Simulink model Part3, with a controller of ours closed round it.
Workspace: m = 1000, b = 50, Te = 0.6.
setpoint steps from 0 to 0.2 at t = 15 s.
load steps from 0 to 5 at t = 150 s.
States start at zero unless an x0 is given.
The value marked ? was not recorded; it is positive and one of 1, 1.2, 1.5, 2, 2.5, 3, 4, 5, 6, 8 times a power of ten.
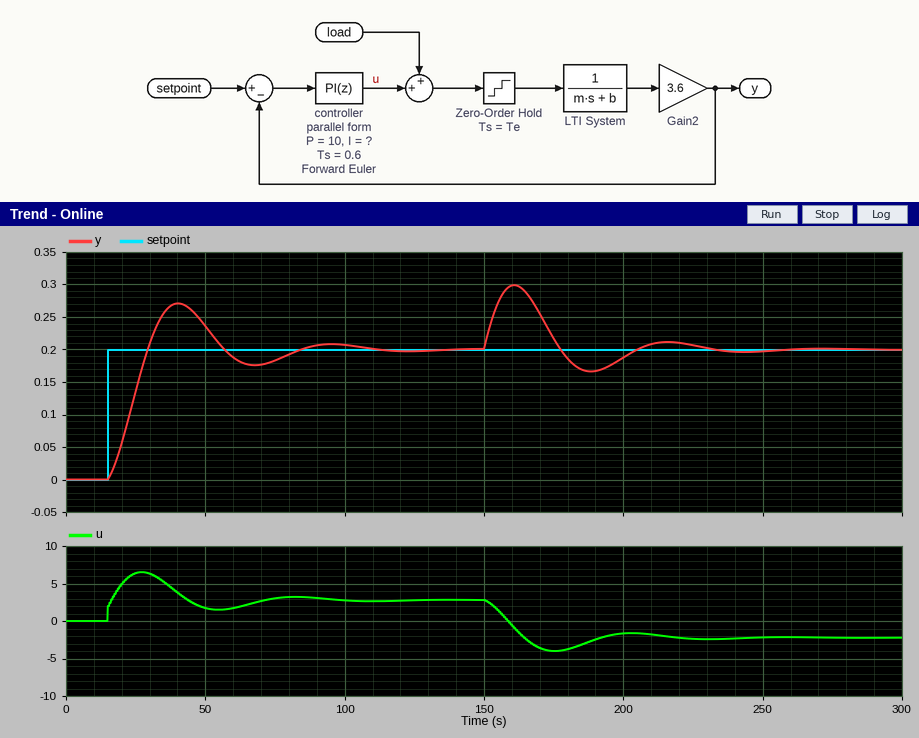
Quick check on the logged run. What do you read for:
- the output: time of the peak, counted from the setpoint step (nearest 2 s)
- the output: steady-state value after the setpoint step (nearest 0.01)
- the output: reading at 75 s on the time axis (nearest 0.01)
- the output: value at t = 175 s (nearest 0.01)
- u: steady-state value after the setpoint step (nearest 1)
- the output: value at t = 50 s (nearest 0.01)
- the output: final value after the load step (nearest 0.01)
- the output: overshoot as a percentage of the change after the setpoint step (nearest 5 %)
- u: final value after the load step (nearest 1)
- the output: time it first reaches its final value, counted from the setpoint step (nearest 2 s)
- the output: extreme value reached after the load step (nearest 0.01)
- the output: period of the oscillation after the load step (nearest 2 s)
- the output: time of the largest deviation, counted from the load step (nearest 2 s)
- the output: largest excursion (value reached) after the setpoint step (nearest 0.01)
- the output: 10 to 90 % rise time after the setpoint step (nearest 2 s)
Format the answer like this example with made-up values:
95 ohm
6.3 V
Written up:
26 s
0.20
0.18
0.22
3
0.24
0.20
35 %
-2
14 s
0.30
56 s
10 s
0.27
10 s
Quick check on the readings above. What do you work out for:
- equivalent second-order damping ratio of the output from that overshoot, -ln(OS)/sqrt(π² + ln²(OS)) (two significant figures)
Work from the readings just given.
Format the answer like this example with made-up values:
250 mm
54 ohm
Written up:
0.32
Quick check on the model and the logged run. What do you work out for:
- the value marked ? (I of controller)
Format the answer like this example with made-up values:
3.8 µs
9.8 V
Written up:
4
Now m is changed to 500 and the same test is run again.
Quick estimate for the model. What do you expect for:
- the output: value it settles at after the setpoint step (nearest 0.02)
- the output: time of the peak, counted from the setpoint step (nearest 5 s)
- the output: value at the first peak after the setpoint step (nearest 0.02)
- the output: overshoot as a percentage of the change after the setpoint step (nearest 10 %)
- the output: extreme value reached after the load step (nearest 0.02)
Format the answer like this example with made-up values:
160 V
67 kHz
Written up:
0.20
20 s
0.24
20 %
0.32
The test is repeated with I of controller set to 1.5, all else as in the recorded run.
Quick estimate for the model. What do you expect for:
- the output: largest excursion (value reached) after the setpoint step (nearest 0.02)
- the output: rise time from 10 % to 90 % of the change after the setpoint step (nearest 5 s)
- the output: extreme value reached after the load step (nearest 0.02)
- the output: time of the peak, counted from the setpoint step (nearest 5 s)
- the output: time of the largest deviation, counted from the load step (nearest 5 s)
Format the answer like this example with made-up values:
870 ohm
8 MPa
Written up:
0.22
20 s
0.32
45 s
15 s
